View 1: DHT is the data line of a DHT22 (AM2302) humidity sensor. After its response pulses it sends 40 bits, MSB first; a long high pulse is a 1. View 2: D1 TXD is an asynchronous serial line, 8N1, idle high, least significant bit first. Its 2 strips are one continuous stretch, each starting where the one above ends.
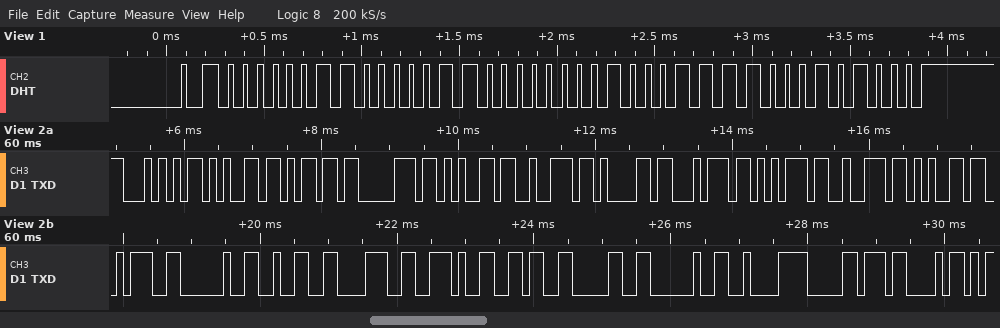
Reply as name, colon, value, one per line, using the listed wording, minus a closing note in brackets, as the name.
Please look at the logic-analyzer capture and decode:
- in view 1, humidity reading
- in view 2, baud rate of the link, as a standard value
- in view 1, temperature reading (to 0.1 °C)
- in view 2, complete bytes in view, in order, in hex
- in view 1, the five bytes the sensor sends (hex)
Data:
in view 1, humidity reading: 77.4 %
in view 2, baud rate of the link, as a standard value: 9600 baud
in view 1, temperature reading: 28.6 °C
in view 2, complete bytes in view, in order, in hex: 54 65 6D 70 65 72 61 74 75 72 65 3A 20 32 38 2E 36 30 20 C2 B0 43
in view 1, the five bytes the sensor sends: 03 06 01 1E 28
